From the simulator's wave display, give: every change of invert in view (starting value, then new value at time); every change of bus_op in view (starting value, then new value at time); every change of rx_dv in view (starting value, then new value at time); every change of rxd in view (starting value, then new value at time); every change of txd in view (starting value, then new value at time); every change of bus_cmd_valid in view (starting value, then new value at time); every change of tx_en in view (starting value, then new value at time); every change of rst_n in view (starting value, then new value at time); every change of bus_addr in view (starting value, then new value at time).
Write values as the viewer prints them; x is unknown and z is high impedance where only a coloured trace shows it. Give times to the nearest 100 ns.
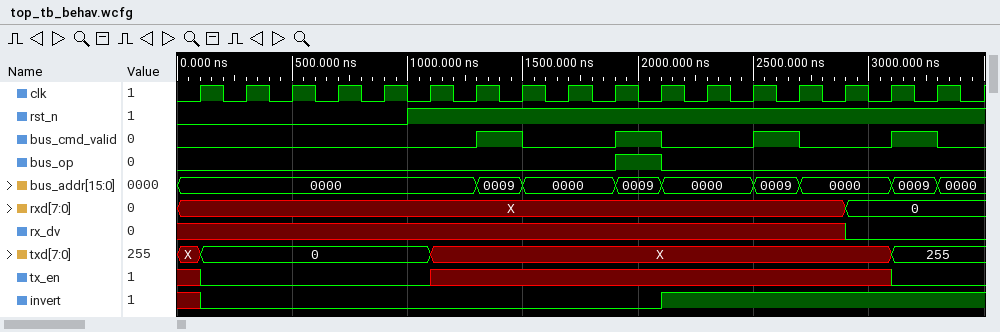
x, 0 at 100 ns, 1 at 2100 ns
0, 1 at 1900 ns, 0 at 2100 ns
x, 0 at 2900 ns
X, 0 at 2900 ns
X, 0 at 100 ns, X at 1100 ns, 255 at 3100 ns
0, 1 at 1300 ns, 0 at 1500 ns, 1 at 1900 ns, 0 at 2100 ns, 1 at 2500 ns, 0 at 2700 ns, 1 at 3100 ns, 0 at 3300 ns
x, 0 at 100 ns, x at 1100 ns, 0 at 3100 ns
0, 1 at 1000 ns
0000, 0009 at 1300 ns, 0000 at 1500 ns, 0009 at 1900 ns, 0000 at 2100 ns, 0009 at 2500 ns, 0000 at 2700 ns, 0009 at 3100 ns, 0000 at 3300 ns
